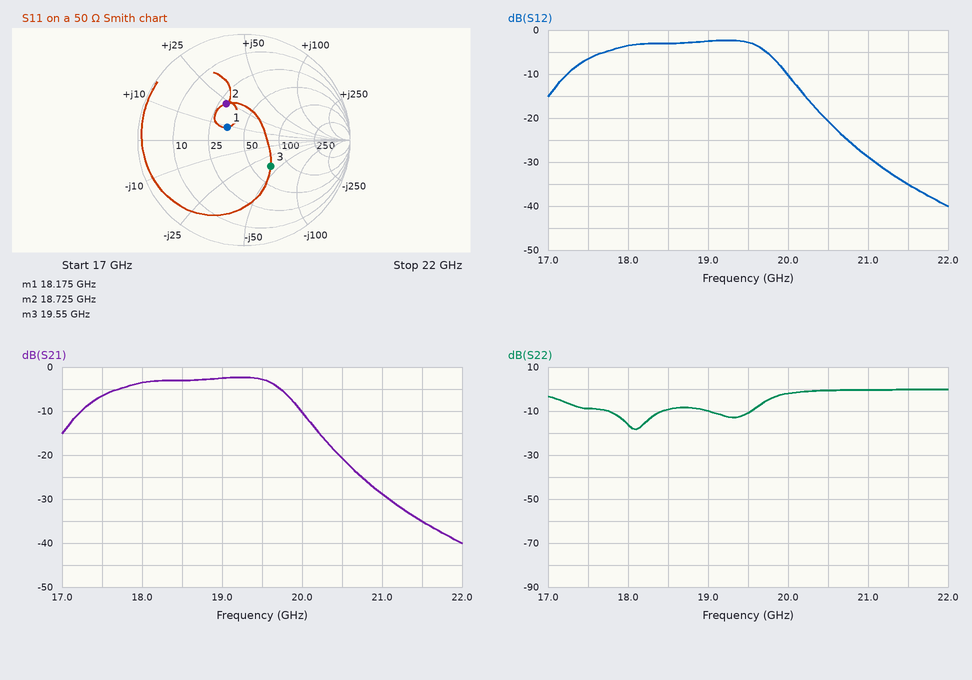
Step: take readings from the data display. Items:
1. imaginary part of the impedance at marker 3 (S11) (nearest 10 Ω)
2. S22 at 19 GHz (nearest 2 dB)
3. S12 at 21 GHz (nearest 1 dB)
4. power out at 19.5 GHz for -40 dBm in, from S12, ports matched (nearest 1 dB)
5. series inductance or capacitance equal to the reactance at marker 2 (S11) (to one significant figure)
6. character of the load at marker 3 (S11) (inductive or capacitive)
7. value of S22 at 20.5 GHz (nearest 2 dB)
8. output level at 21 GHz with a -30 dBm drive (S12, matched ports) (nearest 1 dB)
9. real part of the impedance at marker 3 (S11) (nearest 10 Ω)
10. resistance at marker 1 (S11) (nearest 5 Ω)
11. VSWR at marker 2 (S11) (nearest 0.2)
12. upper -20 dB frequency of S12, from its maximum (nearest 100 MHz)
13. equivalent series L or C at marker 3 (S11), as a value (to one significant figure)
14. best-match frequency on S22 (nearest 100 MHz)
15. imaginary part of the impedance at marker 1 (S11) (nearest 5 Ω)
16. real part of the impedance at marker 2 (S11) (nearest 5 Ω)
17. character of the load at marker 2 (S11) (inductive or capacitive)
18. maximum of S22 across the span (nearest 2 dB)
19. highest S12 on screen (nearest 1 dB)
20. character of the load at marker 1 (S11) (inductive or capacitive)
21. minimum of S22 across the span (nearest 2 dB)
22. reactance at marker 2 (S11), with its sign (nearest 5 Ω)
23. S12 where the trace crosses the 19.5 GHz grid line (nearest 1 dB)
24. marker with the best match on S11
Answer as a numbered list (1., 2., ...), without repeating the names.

1. -40 Ω
2. -10 dB
3. -29 dB
4. -43 dBm
5. 200 pH
6. capacitive
7. 0 dB
8. -59 dBm
9. 70 Ω
10. 35 Ω
11. 2.2
12. 20.6 GHz
13. 200 fF
14. 18.1 GHz
15. +10 Ω
16. 30 Ω
17. inductive
18. 0 dB
19. -2 dB
20. inductive
21. -18 dB
22. +25 Ω
23. -3 dB
24. marker 1
